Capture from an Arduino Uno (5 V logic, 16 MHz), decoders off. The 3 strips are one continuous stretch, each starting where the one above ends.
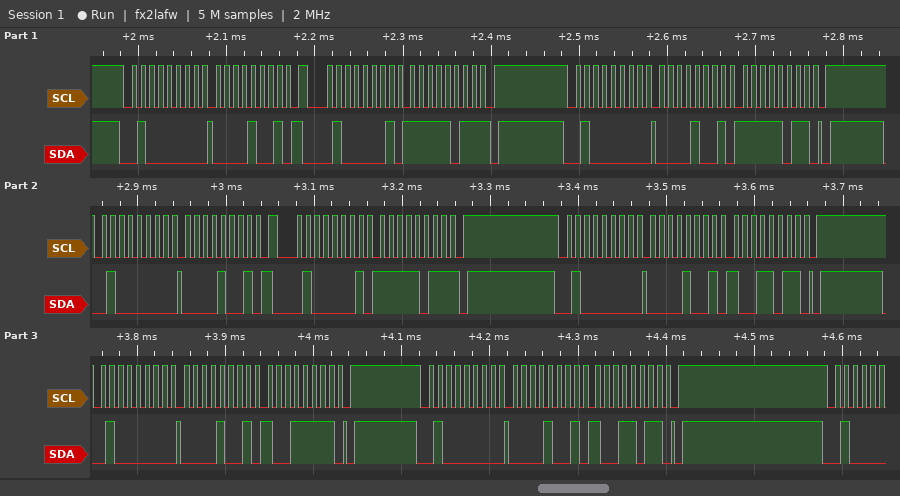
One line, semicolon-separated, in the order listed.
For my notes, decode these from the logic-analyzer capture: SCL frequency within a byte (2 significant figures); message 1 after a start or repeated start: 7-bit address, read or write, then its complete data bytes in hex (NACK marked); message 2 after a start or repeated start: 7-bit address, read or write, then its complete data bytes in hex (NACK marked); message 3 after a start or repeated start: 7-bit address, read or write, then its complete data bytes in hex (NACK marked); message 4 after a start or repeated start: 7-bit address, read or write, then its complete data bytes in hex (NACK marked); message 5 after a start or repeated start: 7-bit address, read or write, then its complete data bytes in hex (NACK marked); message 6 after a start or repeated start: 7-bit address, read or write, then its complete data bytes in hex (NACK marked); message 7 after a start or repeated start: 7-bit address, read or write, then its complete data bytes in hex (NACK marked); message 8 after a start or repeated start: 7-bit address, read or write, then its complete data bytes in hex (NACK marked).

100 kHz; 0x20 write: 09; 0x20 read: FB NACK; 0x20 write: 09 FB; 0x20 write: 09; 0x20 read: FB NACK; 0x20 write: 09 9B; 0x20 write: 09 9F; 0x20 write: 09 9B
